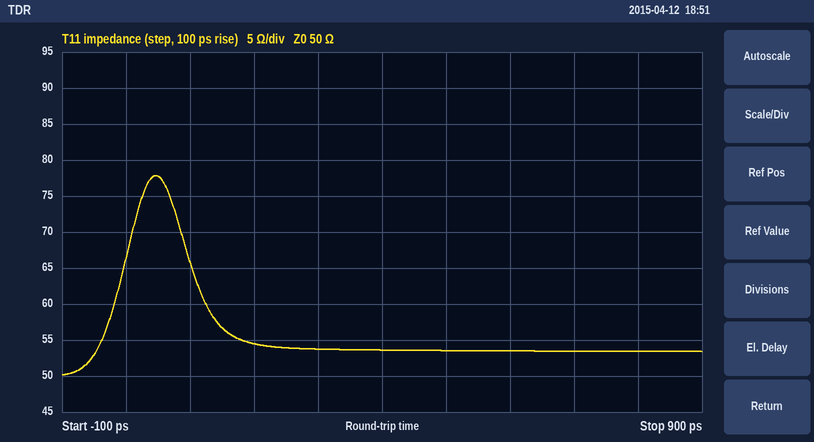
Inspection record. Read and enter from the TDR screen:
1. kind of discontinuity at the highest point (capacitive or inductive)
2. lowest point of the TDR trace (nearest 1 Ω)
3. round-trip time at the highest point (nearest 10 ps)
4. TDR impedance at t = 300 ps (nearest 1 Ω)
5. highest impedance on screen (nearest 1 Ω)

inductive
50 Ω
50 ps
54 Ω
78 Ω
